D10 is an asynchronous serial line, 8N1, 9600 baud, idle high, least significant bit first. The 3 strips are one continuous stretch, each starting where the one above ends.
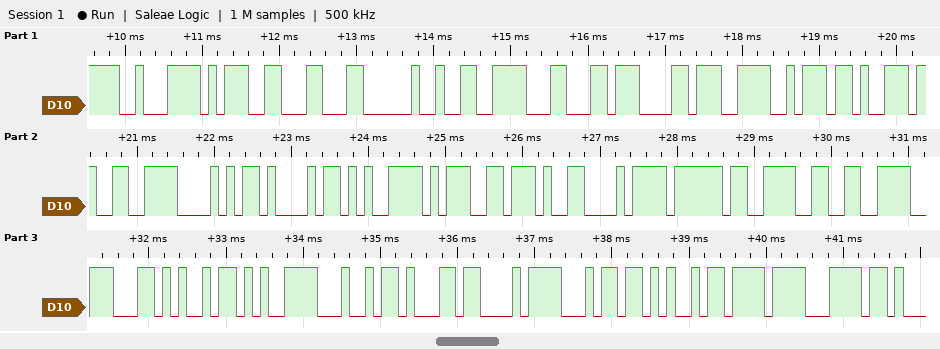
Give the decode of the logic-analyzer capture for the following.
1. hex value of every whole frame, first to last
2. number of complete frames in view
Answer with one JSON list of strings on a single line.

["E2 9D 8C 20 E6 8C 87 E7 BA B9 E6 A8 A1 E5 9D 97 E8 BF 9E E6 8E A5 E5 A4 B1 E8 B4 A5 EF BC", "30"]
